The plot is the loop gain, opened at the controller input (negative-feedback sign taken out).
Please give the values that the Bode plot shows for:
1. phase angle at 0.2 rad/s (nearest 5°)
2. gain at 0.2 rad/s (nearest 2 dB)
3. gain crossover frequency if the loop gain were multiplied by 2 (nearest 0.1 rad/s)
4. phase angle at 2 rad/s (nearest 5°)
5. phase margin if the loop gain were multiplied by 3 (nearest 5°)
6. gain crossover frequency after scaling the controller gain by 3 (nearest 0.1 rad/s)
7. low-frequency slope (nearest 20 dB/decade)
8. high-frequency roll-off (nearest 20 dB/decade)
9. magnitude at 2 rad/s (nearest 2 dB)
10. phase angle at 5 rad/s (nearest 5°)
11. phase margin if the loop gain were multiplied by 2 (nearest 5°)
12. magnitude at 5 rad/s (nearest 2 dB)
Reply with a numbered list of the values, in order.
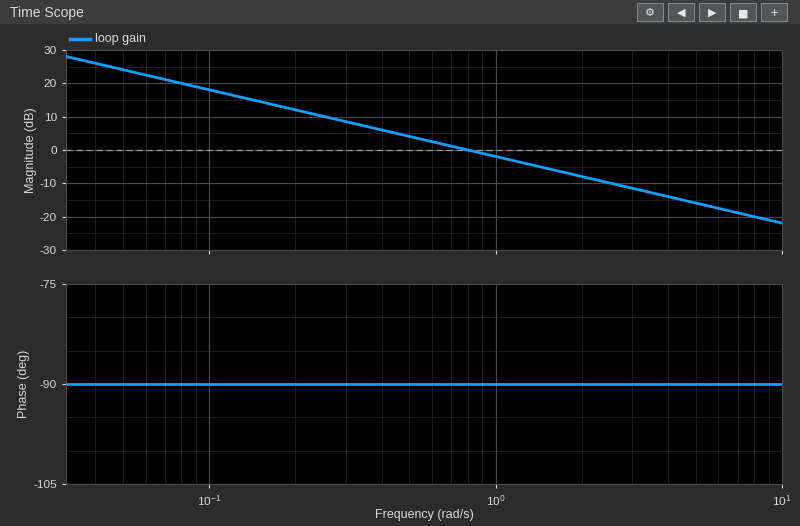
1. -90°
2. 12 dB
3. 1.6 rad/s
4. -90°
5. 90°
6. 2.4 rad/s
7. -20 dB/decade
8. -20 dB/decade
9. -8 dB
10. -90°
11. 90°
12. -16 dB
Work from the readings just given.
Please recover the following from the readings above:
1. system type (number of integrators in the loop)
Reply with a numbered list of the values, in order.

1. 1
